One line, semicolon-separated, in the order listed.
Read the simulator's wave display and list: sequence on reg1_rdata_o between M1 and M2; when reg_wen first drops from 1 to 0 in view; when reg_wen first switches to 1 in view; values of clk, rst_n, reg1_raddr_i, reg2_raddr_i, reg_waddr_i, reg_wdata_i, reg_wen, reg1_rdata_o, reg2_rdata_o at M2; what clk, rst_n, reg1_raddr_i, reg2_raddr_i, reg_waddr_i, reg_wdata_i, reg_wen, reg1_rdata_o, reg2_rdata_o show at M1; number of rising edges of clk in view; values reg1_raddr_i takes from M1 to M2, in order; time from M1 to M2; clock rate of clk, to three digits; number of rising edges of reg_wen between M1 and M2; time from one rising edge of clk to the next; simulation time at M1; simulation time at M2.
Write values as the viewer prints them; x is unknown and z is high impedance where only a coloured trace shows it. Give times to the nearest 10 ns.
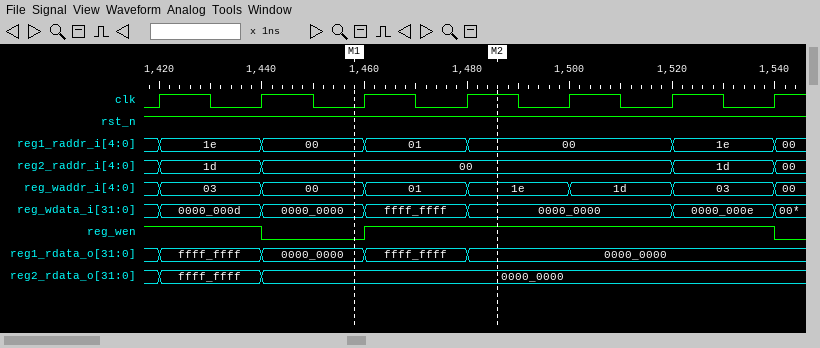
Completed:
0000_0000, ffff_ffff, 0000_0000; 1440 ns; 1460 ns; clk=1, rst_n=1, reg1_raddr_i=00, reg2_raddr_i=00, reg_waddr_i=1e, reg_wdata_i=0000_0000, reg_wen=1, reg1_rdata_o=0000_0000, reg2_rdata_o=0000_0000; clk=0, rst_n=1, reg1_raddr_i=00, reg2_raddr_i=00, reg_waddr_i=00, reg_wdata_i=0000_0000, reg_wen=0, reg1_rdata_o=0000_0000, reg2_rdata_o=0000_0000; 7; 00, 01, 00; 30 ns; 50.0 MHz; 1; 20 ns; 1460 ns; 1490 ns
